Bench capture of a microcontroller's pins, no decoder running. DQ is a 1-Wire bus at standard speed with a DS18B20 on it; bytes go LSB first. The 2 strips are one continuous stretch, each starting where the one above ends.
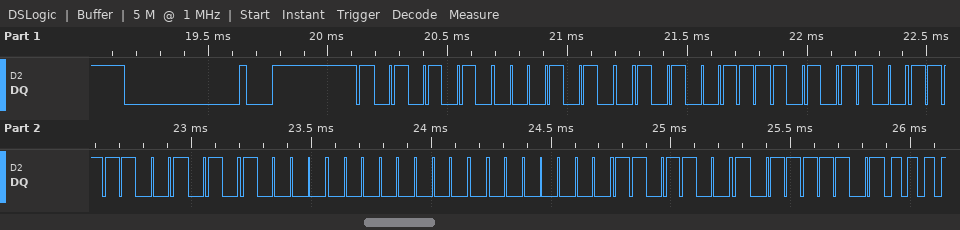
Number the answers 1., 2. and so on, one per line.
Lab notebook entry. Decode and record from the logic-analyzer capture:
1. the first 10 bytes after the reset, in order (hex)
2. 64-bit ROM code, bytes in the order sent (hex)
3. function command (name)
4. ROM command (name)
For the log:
1. 55 28 E5 35 9F 0A 00 00 9B BE
2. 28 E5 35 9F 0A 00 00 9B
3. Read Scratchpad
4. Match ROM
